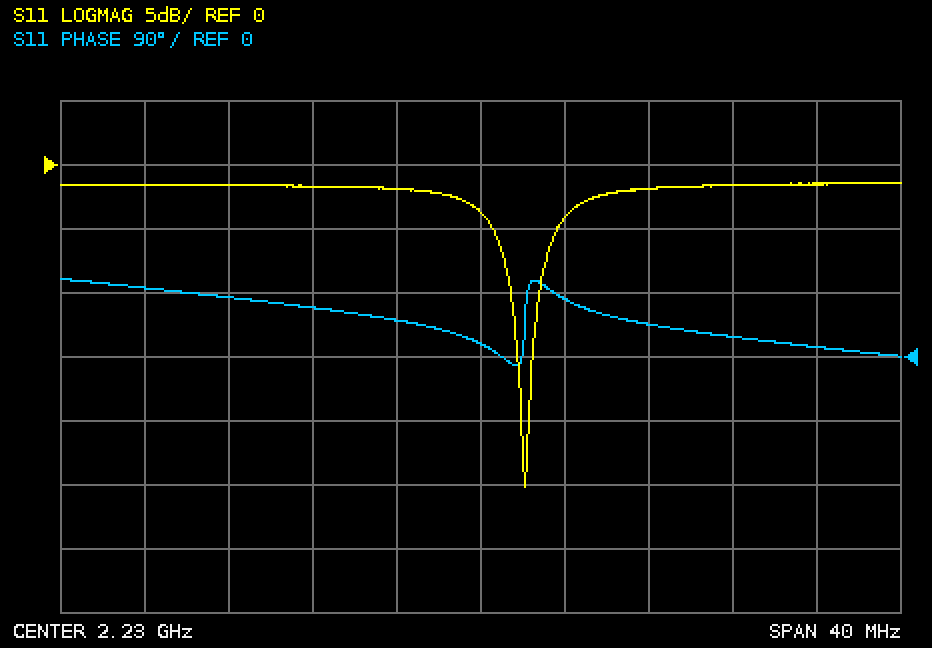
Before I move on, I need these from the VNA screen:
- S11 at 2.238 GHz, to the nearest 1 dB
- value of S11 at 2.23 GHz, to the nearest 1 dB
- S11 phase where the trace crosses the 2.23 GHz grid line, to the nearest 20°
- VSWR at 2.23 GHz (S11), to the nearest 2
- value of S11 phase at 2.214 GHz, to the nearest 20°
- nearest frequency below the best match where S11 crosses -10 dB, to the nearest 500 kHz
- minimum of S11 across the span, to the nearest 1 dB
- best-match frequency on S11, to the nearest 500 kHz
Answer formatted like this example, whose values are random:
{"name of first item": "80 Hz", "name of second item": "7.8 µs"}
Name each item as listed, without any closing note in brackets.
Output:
{"S11 at 2.238 GHz, to the nearest 1 dB": "-2 dB", "value of S11 at 2.23 GHz, to the nearest 1 dB": "-4 dB", "S11 phase where the trace crosses the 2.23 GHz grid line, to the nearest 20°": "20°", "VSWR at 2.23 GHz (S11), to the nearest 2": "4", "value of S11 phase at 2.214 GHz, to the nearest 20°": "100°", "nearest frequency below the best match where S11 crosses -10 dB, to the nearest 500 kHz": "2.2315 GHz", "minimum of S11 across the span, to the nearest 1 dB": "-25 dB", "best-match frequency on S11, to the nearest 500 kHz": "2.2320 GHz"}
